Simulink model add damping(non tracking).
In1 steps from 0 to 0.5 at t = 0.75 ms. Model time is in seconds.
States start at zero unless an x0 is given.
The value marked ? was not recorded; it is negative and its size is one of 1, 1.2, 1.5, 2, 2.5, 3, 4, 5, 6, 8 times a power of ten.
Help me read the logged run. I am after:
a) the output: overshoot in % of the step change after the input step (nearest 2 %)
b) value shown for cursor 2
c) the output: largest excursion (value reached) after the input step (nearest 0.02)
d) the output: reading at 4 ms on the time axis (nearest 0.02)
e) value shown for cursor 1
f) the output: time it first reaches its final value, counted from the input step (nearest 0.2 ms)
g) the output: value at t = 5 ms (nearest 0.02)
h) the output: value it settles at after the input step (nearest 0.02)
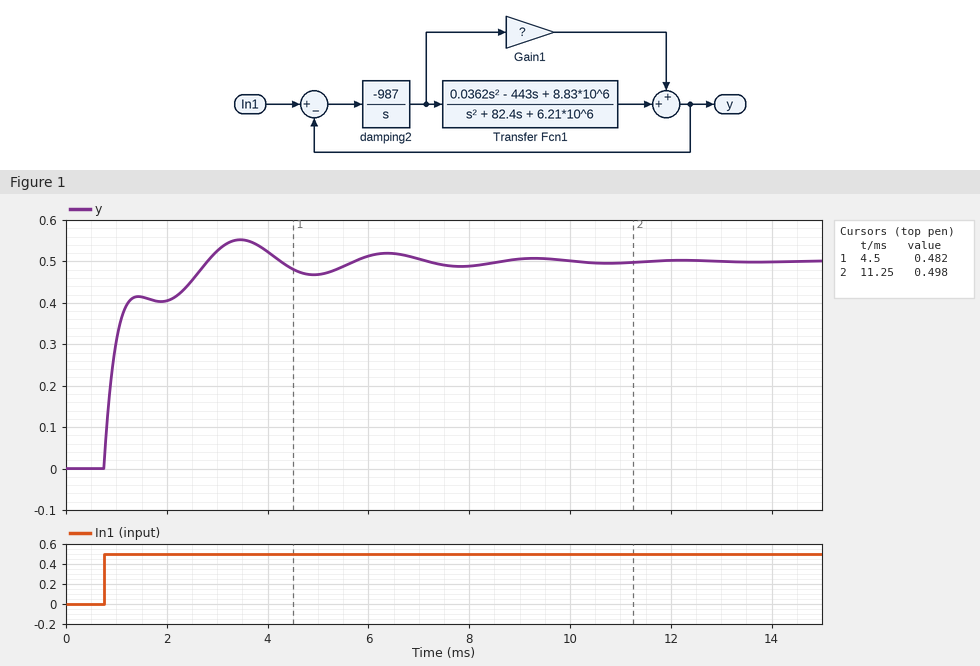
10 %
0.498
0.56
0.52
0.482
2.0 ms
0.46
0.50
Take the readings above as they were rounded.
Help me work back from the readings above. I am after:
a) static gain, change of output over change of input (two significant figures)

1.0
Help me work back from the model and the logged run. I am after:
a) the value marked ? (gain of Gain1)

-4
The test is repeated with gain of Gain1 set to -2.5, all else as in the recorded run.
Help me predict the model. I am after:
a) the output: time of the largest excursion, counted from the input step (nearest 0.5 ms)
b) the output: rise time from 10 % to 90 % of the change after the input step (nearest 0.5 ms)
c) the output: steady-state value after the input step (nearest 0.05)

3.0 ms
2.5 ms
0.50
